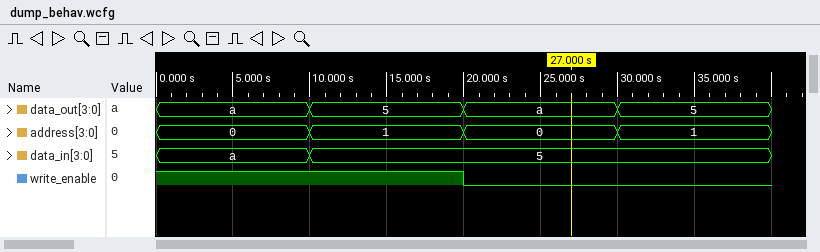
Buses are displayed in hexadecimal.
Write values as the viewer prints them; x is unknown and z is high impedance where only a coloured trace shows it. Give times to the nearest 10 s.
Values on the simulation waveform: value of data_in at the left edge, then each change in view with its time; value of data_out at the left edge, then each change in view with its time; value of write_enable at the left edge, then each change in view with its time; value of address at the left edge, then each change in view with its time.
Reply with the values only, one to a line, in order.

a, 5 at 10 s
a, 5 at 10 s, a at 20 s, 5 at 30 s
1, 0 at 20 s
0, 1 at 10 s, 0 at 20 s, 1 at 30 s
